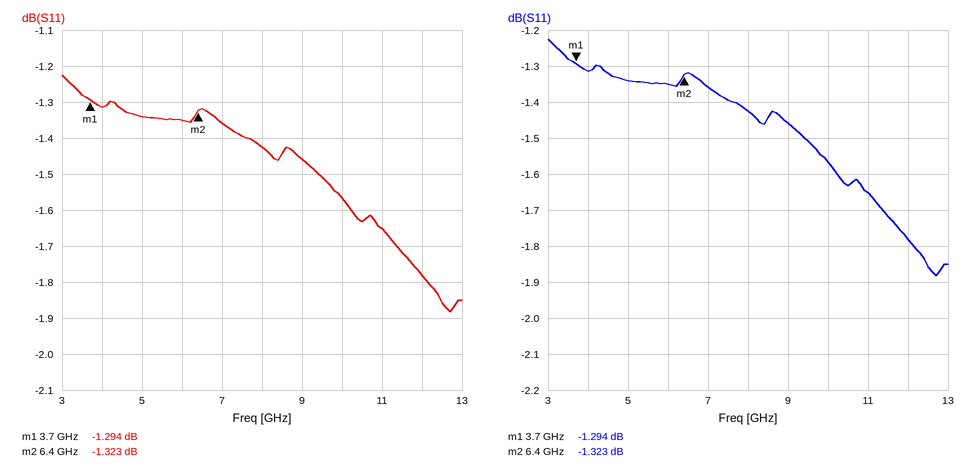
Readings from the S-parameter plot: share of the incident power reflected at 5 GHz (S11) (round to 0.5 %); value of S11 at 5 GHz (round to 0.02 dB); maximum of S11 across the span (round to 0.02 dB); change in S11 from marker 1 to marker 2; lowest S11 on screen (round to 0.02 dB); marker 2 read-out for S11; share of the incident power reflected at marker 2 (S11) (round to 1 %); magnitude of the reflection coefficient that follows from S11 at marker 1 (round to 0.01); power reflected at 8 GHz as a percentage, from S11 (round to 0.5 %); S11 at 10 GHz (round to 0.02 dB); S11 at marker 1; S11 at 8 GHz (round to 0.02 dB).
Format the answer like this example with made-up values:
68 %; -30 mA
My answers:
73.5 %; -1.34 dB; -1.22 dB; -0.029 dB; -1.88 dB; -1.323 dB; 74 %; 0.86; 72.0 %; -1.56 dB; -1.294 dB; -1.42 dB
